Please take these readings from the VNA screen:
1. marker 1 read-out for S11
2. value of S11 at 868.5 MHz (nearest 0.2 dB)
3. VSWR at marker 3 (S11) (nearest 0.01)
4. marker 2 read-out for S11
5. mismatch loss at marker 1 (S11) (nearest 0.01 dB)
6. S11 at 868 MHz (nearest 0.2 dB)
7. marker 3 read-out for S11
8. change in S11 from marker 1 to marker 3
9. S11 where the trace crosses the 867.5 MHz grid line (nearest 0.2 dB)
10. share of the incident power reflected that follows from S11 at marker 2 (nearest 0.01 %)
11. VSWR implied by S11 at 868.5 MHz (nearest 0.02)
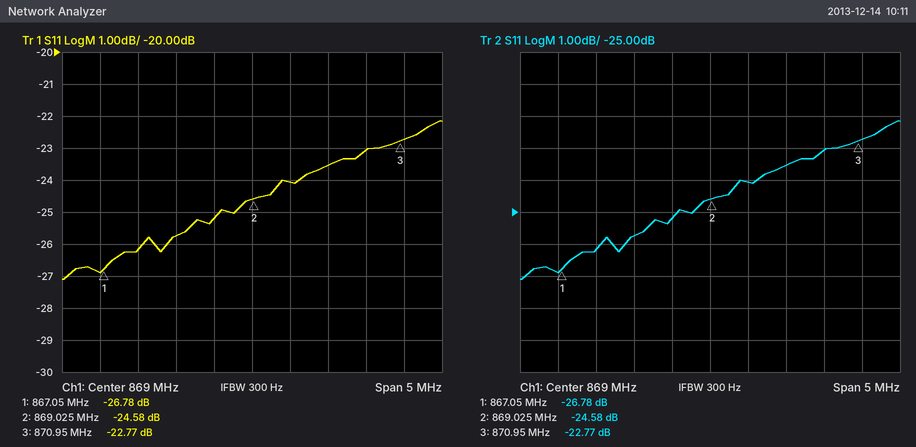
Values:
-26.78 dB
-25.2 dB
1.16
-24.58 dB
0.01 dB
-25.8 dB
-22.77 dB
4.01 dB
-26.2 dB
0.35 %
1.12
